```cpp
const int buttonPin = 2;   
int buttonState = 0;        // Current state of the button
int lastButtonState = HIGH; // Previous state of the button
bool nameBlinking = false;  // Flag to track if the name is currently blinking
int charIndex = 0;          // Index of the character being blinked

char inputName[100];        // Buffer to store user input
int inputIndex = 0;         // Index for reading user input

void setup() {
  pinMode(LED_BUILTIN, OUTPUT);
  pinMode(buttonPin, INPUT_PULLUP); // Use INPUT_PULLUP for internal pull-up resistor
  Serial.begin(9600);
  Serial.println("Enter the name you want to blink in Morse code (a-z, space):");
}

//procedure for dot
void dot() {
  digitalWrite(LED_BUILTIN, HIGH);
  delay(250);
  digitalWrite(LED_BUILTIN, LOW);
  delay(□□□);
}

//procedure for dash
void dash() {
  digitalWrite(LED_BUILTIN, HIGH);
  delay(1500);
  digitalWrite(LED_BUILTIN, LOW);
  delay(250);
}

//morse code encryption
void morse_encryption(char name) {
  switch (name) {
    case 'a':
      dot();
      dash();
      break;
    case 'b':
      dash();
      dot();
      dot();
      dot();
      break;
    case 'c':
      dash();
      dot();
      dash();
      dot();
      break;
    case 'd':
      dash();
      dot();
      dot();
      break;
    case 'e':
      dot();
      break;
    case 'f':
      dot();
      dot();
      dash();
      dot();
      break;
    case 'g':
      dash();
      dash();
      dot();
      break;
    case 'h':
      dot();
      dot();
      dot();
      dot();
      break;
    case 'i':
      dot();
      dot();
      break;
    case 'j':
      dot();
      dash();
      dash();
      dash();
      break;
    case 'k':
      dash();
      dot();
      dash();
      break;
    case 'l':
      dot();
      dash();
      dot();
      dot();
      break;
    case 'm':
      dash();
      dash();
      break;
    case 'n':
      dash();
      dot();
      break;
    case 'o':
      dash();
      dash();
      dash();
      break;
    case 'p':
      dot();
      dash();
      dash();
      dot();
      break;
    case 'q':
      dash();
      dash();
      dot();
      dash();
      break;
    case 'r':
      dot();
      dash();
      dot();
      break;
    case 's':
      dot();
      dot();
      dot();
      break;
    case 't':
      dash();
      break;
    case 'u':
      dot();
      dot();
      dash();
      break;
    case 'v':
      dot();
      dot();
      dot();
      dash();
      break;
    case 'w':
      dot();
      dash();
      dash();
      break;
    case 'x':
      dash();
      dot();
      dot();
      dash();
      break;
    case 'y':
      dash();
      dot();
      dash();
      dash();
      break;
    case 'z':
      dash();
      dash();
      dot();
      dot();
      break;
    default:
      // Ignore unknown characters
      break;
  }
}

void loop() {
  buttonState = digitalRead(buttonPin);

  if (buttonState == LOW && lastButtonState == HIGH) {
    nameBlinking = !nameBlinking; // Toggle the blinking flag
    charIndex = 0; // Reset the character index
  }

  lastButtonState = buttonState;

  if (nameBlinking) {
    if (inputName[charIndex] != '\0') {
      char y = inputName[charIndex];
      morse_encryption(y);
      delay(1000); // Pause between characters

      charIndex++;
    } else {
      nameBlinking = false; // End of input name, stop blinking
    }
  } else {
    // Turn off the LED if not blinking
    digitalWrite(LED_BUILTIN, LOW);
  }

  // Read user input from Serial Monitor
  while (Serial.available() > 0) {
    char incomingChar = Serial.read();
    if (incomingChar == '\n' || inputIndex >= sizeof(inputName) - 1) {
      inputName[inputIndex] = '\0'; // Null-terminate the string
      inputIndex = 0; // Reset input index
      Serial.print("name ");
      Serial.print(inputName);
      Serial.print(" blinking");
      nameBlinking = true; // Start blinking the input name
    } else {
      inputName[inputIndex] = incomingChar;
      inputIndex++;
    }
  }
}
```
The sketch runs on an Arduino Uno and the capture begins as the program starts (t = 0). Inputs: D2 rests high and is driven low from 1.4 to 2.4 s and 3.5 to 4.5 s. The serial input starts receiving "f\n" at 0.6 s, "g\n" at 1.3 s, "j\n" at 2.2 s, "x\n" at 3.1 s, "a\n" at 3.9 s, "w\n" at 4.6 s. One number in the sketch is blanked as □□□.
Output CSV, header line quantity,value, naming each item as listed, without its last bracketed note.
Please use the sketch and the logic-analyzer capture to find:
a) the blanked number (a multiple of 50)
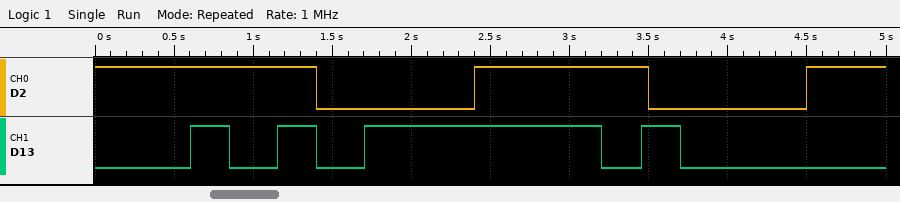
quantity,value
the blanked number,300
